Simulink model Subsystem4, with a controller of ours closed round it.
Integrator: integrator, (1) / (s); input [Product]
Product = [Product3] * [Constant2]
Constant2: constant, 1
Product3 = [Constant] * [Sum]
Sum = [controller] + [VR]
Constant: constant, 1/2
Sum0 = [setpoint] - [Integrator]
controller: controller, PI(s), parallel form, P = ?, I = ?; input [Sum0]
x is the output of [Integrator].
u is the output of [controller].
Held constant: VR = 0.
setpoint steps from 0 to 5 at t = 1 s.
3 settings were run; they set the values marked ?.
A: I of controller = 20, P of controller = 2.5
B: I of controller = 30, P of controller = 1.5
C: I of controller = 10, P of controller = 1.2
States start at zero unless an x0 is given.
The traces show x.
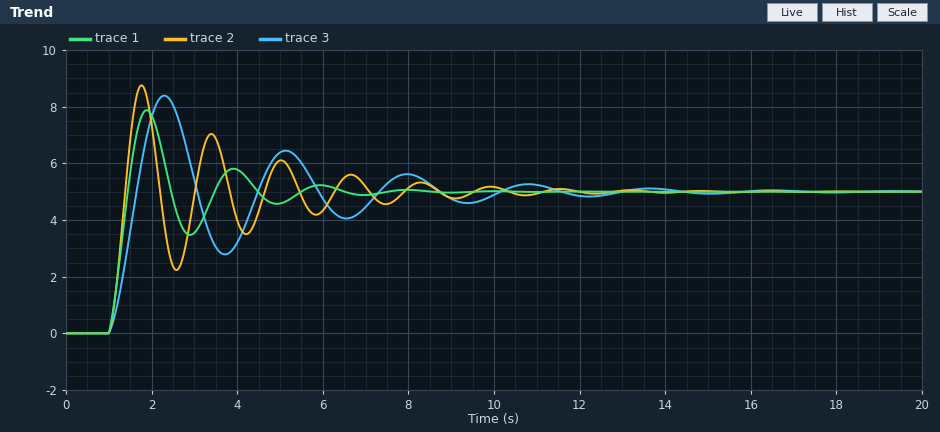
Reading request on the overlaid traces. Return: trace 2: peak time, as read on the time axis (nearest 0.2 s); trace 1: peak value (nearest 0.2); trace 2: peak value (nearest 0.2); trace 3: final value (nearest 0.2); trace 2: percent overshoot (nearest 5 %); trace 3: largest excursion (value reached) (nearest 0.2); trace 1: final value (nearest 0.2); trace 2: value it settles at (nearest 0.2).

1.8 s
7.8
8.8
5.0
75 %
8.4
5.0
5.0
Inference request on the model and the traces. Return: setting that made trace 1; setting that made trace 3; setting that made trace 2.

A
C
B
